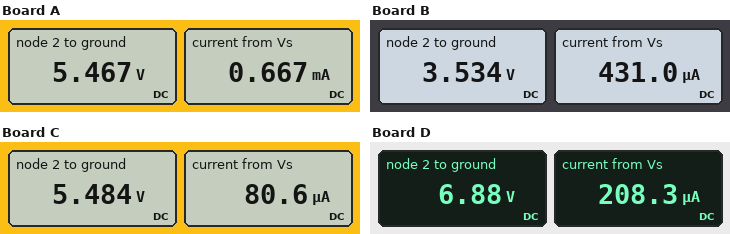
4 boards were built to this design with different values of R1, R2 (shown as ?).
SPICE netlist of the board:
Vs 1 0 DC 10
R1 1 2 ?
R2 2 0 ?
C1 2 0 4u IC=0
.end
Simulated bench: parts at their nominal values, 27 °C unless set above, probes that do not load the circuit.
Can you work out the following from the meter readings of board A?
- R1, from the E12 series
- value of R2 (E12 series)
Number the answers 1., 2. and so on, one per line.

1. 6.8 kΩ
2. 8.2 kΩ
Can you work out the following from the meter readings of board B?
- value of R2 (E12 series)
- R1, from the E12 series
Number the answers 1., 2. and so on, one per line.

1. 8.2 kΩ
2. 15 kΩ
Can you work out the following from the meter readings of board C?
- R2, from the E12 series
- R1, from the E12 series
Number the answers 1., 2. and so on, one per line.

1. 68 kΩ
2. 56 kΩ
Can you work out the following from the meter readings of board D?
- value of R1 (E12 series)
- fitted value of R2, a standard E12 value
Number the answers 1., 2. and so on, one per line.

1. 15 kΩ
2. 33 kΩ
